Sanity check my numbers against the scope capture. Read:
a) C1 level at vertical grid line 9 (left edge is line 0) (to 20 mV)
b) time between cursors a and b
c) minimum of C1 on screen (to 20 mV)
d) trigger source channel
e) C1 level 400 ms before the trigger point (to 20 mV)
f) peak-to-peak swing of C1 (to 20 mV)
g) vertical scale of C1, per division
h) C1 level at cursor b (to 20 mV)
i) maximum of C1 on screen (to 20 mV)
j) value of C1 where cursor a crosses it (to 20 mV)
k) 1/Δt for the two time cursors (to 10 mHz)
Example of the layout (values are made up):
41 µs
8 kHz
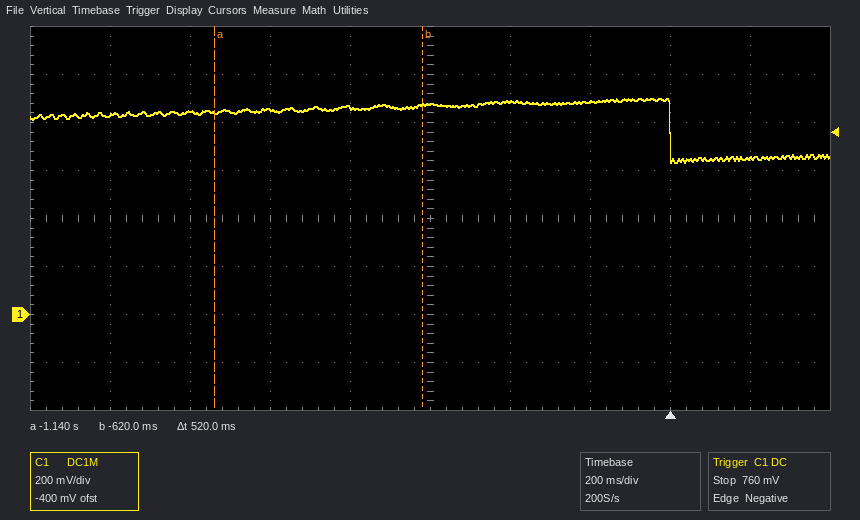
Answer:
660 mV
520 ms
640 mV
C1
880 mV
260 mV
200 mV
880 mV
900 mV
840 mV
1.92 Hz
